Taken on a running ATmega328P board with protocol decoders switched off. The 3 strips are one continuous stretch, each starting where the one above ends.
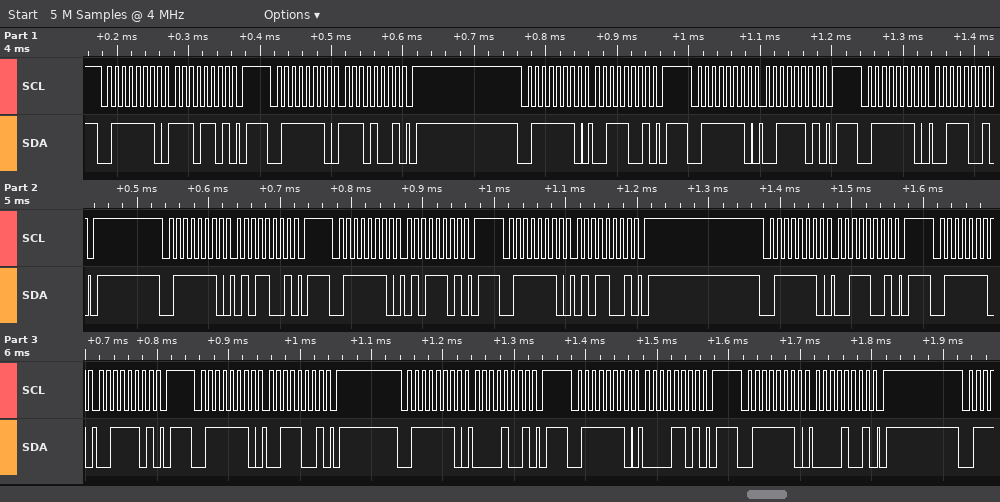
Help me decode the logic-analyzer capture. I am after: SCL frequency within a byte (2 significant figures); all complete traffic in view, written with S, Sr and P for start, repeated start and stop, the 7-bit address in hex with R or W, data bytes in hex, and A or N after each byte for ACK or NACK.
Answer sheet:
100 kHz
S 3FW A ED A P S 3FW A E9 A P S 3FW A 39 A P S 3FW A 3D A P S 3FW A 39 A P S 3FW A 59 A P S 3FW A 5D A P S 3FW A 59 A P S 3FW A 39 A P S 3FW A 3D A P S 3FW A 39 A P S 3FW A 09 A P S 3FW A 0D A P S 3FW A 09 A P
